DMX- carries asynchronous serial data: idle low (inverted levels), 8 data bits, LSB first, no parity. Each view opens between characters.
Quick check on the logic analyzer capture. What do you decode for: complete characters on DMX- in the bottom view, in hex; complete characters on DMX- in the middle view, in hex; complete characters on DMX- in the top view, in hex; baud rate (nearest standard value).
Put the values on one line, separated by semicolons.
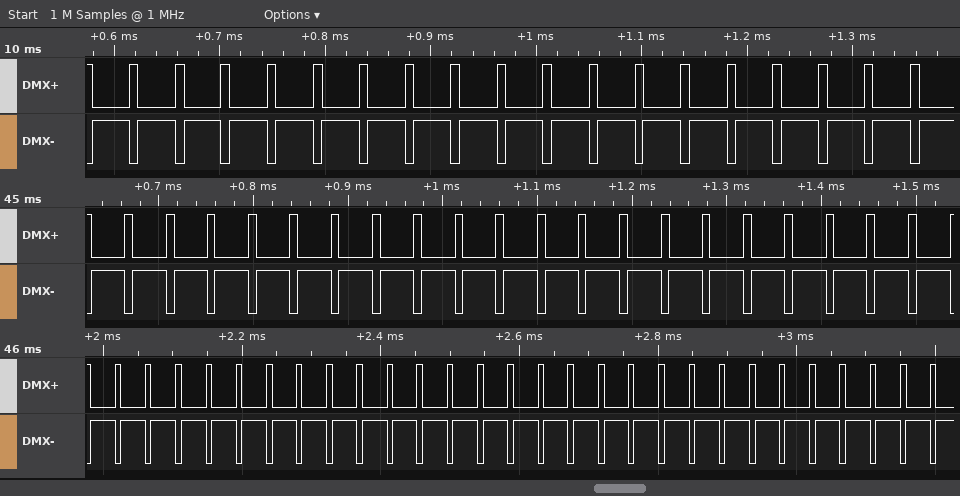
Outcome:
08, 08, 08, 08, 08, 08, 08, 08, 08, 08, 08, 08, 08, 08; 08, 08, 08, 08, 08, 08, 08, 08, 08, 08; 08, 08, 08, 08, 08, 08, 08, 08, 08; 115200 baud
